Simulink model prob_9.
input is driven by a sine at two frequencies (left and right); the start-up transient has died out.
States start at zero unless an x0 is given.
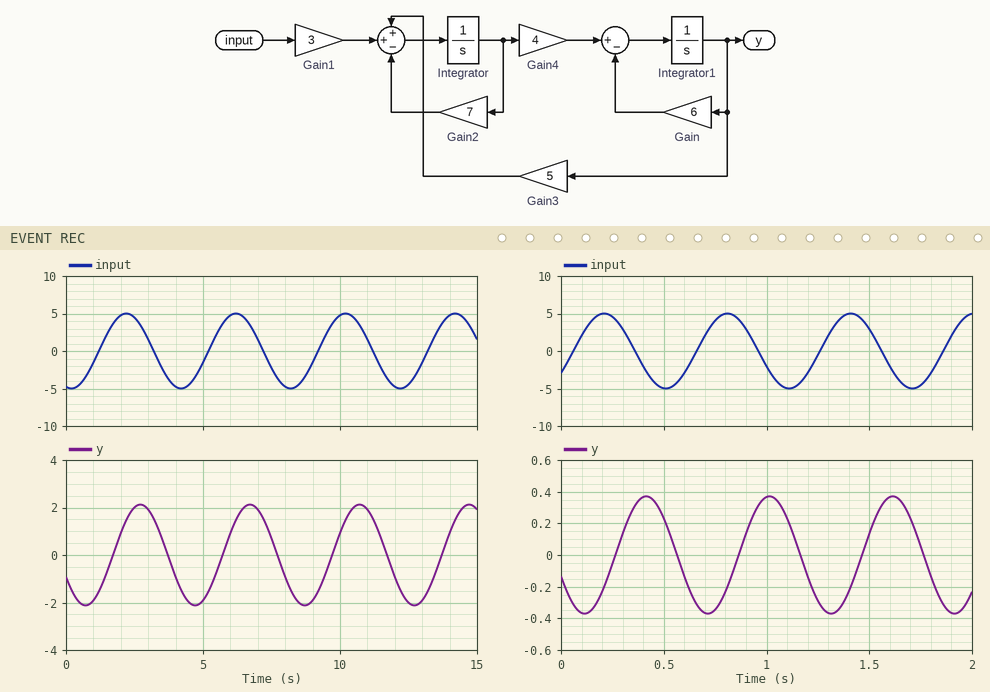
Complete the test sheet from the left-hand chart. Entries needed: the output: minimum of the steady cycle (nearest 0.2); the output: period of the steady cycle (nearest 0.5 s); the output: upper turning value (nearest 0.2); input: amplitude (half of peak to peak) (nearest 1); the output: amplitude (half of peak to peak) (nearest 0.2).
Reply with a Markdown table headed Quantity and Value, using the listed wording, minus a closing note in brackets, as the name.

| Quantity | Value |
|---|---|
| the output: minimum of the steady cycle | -2.2 |
| the output: period of the steady cycle | 4.0 s |
| the output: upper turning value | 2.2 |
| input: amplitude (half of peak to peak) | 5 |
| the output: amplitude (half of peak to peak) | 2.2 |
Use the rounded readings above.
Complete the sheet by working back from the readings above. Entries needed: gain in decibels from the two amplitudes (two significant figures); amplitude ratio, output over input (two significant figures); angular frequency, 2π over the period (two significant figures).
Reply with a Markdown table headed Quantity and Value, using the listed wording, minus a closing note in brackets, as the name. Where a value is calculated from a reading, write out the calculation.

| Quantity | Value |
|---|---|
| gain in decibels from the two amplitudes | 20 log10(2.2 / 5) = -7.1 dB |
| amplitude ratio, output over input | 2.2 / 5 = 0.44 |
| angular frequency, 2π over the period | 2π / 4 = 1.6 rad/s |
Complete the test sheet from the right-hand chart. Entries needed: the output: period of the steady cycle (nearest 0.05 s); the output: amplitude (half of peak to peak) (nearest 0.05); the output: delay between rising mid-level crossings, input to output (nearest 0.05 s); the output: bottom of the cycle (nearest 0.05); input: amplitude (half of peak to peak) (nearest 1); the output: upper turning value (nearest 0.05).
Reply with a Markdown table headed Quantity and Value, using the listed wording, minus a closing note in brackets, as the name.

| Quantity | Value |
|---|---|
| the output: period of the steady cycle | 0.60 s |
| the output: amplitude (half of peak to peak) | 0.35 |
| the output: delay between rising mid-level crossings, input to output | 0.20 s |
| the output: bottom of the cycle | -0.35 |
| input: amplitude (half of peak to peak) | 5 |
| the output: upper turning value | 0.35 |
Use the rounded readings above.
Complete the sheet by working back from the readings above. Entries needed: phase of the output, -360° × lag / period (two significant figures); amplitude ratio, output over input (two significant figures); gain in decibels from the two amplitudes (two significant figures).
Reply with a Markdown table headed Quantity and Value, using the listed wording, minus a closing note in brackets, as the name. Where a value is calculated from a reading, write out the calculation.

| Quantity | Value |
|---|---|
| phase of the output, -360° × lag / period | -360 × 0.2 / 0.6 = -120° |
| amplitude ratio, output over input | 0.35 / 5 = 0.070 |
| gain in decibels from the two amplitudes | 20 log10(0.35 / 5) = -23 dB |
